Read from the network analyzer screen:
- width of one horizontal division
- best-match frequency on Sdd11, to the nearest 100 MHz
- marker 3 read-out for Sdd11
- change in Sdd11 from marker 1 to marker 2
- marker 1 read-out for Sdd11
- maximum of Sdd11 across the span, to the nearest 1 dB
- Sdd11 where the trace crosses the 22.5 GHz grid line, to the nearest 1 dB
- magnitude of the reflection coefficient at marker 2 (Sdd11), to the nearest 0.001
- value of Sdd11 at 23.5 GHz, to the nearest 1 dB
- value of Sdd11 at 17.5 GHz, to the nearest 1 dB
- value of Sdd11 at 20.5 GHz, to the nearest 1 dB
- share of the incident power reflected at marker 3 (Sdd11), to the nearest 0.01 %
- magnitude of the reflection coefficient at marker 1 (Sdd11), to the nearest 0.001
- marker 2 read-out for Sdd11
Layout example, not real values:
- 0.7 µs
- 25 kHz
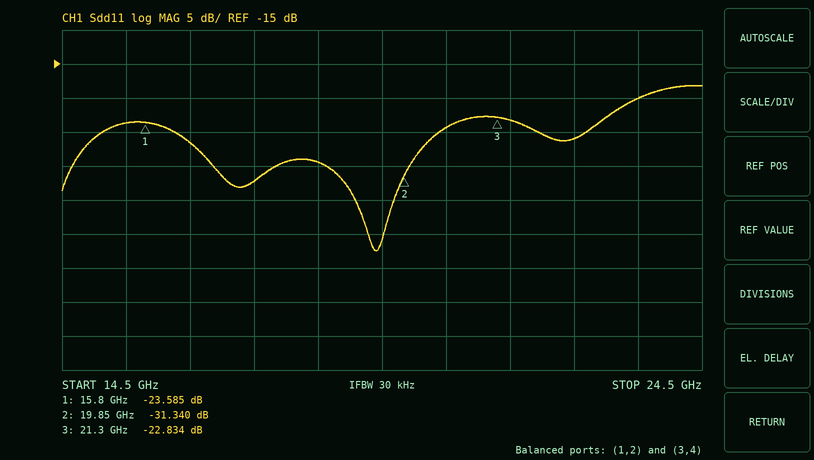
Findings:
- 1 GHz
- 19.4 GHz
- -22.834 dB
- -7.755 dB
- -23.585 dB
- -18 dB
- -26 dB
- 0.027
- -20 dB
- -32 dB
- -24 dB
- 0.52 %
- 0.066
- -31.340 dB
